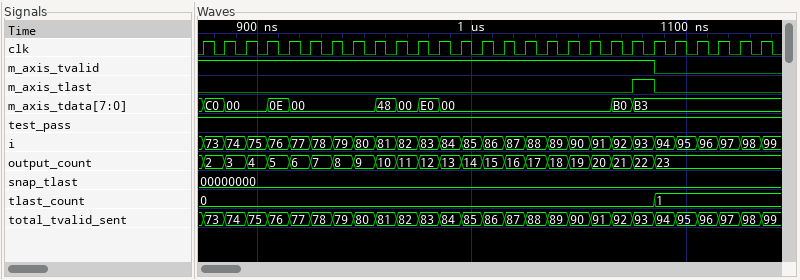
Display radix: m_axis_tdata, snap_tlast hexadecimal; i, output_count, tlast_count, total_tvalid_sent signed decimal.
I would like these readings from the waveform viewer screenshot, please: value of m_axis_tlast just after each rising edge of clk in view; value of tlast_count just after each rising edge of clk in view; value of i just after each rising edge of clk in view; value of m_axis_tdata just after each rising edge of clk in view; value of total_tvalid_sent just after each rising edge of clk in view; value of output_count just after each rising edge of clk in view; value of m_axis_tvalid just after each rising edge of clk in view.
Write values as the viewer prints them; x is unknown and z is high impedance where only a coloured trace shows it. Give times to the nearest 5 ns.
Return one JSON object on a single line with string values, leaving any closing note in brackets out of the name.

{"value of m_axis_tlast just after each rising edge of clk in view": "0 0 0 0 0 0 0 0 0 0 0 0 0 0 0 0 0 0 0 0 1 0 0 0 0 0 0", "value of tlast_count just after each rising edge of clk in view": "0, 0, 0, 0, 0, 0, 0, 0, 0, 0, 0, 0, 0, 0, 0, 0, 0, 0, 0, 0, 0, 1, 1, 1, 1, 1, 1", "value of i just after each rising edge of clk in view": "73, 74, 75, 76, 77, 78, 79, 80, 81, 82, 83, 84, 85, 86, 87, 88, 89, 90, 91, 92, 93, 94, 95, 96, 97, 98, 99", "value of m_axis_tdata just after each rising edge of clk in view": "C0, 00, 00, 0E, 00, 00, 00, 00, 48, 00, E0, 00, 00, 00, 00, 00, 00, 00, 00, B0, B3, B3, B3, B3, B3, B3, B3", "value of total_tvalid_sent just after each rising edge of clk in view": "73, 74, 75, 76, 77, 78, 79, 80, 81, 82, 83, 84, 85, 86, 87, 88, 89, 90, 91, 92, 93, 94, 95, 96, 97, 98, 99", "value of output_count just after each rising edge of clk in view": "2, 3, 4, 5, 6, 7, 8, 9, 10, 11, 12, 13, 14, 15, 16, 17, 18, 19, 20, 21, 22, 23, 23, 23, 23, 23, 23", "value of m_axis_tvalid just after each rising edge of clk in view": "1 1 1 1 1 1 1 1 1 1 1 1 1 1 1 1 1 1 1 1 1 0 0 0 0 0 0"}
